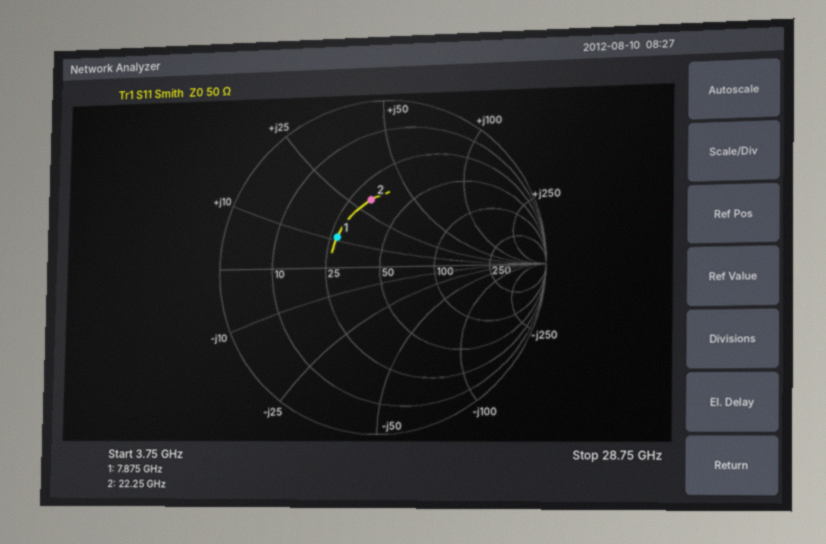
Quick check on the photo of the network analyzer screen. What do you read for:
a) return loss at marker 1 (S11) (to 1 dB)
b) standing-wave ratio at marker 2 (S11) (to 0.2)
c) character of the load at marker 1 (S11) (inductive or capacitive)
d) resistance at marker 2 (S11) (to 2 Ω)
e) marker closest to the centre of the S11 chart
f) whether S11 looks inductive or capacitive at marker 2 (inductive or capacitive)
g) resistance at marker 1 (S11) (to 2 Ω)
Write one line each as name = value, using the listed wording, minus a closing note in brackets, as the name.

return loss at marker 1 (S11) = 10 dB
standing-wave ratio at marker 2 (S11) = 2.4
character of the load at marker 1 (S11) = inductive
resistance at marker 2 (S11) = 32 Ω
marker closest to the centre of the S11 chart = marker 1
whether S11 looks inductive or capacitive at marker 2 = inductive
resistance at marker 1 (S11) = 28 Ω
